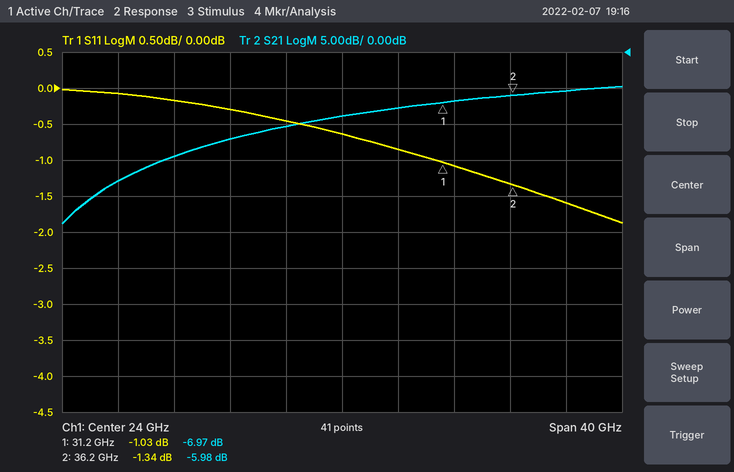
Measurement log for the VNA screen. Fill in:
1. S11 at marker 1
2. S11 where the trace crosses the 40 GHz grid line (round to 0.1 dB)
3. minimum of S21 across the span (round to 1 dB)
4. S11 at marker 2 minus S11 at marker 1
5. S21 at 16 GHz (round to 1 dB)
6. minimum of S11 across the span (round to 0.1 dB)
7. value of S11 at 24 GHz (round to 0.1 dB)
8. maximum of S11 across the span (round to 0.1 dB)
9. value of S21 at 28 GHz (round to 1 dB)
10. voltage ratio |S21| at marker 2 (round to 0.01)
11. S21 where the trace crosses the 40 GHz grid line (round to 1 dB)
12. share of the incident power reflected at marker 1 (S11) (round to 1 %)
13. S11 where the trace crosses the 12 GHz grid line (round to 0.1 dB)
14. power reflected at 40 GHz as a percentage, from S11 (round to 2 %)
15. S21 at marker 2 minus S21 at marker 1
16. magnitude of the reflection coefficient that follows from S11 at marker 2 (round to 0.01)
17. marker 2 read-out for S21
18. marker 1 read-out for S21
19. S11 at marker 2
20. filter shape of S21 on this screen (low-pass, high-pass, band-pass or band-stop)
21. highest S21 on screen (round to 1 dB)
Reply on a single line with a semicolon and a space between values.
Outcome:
-1.03 dB; -1.6 dB; -24 dB; -0.31 dB; -12 dB; -1.9 dB; -0.6 dB; 0.0 dB; -8 dB; 0.50; -5 dB; 79 %; -0.2 dB; 70 %; 0.99 dB; 0.86; -5.98 dB; -6.97 dB; -1.34 dB; high-pass; -5 dB
